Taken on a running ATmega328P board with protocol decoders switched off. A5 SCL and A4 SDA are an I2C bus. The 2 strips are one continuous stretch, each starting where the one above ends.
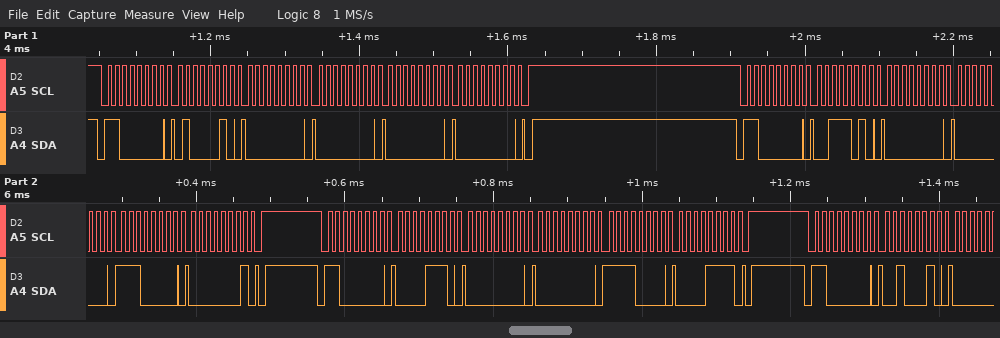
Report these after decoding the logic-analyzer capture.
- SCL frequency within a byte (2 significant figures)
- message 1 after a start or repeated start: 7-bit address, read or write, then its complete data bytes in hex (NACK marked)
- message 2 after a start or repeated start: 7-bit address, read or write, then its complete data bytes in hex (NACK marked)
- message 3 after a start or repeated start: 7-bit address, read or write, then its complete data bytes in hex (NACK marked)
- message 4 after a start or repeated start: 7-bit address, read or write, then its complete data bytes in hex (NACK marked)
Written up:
100 kHz
0x60 write: 42 00 00 00 00
0x60 write: 3A 00 00 E0 01
0x60 write: 0E 00 00 F0 0F
0x60 write: 22
